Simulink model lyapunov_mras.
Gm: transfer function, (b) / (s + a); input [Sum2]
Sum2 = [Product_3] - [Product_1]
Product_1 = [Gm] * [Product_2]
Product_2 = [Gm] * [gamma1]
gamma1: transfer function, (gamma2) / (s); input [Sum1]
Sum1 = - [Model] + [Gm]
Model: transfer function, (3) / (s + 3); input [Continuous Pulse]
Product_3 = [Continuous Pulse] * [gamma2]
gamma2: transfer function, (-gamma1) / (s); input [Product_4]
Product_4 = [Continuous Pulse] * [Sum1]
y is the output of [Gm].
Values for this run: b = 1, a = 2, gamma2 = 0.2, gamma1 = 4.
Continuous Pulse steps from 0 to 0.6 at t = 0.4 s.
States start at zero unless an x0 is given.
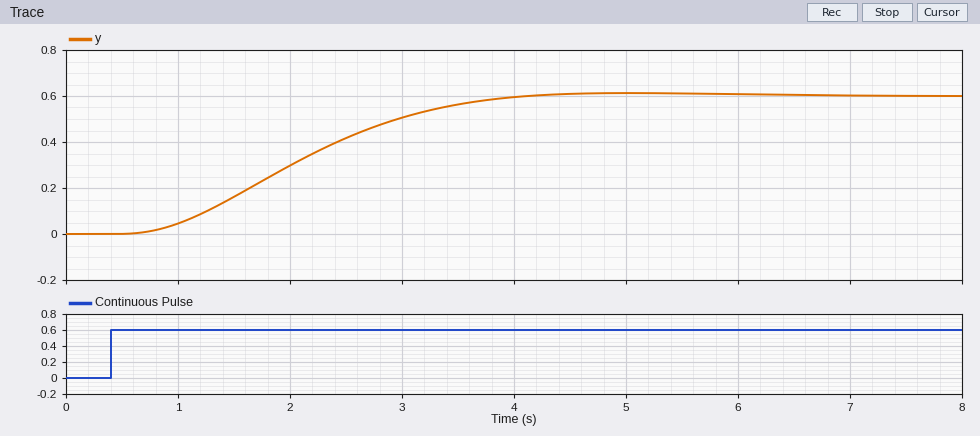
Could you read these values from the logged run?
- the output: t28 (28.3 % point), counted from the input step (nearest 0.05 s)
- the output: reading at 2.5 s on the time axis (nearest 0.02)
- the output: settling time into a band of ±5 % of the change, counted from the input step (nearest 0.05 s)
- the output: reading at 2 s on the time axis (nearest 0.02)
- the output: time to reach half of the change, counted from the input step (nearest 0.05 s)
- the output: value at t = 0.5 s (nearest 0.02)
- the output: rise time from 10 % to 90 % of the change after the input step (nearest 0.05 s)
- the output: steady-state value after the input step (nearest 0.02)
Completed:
1.15 s
0.42
3.20 s
0.30
1.60 s
0.00
2.20 s
0.60
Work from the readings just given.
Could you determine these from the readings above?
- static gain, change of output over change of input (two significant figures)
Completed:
1.0
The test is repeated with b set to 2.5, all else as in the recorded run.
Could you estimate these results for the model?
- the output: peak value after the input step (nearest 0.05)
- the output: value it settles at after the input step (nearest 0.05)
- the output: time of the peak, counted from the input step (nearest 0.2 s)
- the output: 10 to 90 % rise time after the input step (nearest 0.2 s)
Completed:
0.70
0.60
2.4 s
1.0 s
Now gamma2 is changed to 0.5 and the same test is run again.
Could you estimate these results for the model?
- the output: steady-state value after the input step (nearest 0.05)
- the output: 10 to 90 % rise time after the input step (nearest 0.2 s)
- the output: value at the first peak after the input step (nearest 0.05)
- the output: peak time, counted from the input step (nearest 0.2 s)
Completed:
0.60
2.0 s
0.65
4.2 s
